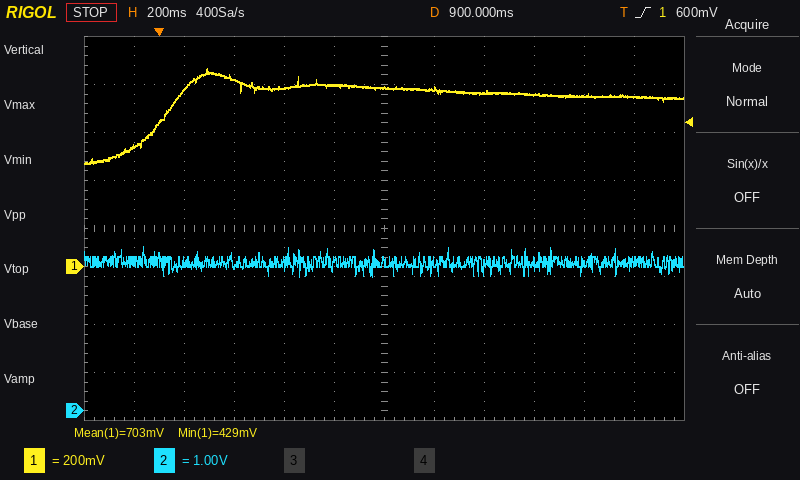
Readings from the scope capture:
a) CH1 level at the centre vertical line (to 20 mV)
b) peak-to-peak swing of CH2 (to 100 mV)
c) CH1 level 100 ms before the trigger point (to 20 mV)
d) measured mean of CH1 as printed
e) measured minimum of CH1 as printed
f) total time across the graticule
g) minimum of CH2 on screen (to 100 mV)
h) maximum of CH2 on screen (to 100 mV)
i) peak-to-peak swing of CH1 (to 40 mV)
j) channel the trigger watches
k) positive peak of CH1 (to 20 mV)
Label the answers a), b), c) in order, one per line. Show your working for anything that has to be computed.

a) 740 mV
b) 3.4 V − (2.8 V) = 600 mV
c) 500 mV
d) 703 mV
e) 429 mV
f) 2.4 s
g) 2.8 V
h) 3.4 V
i) 400 mV
j) CH1
k) 820 mV
